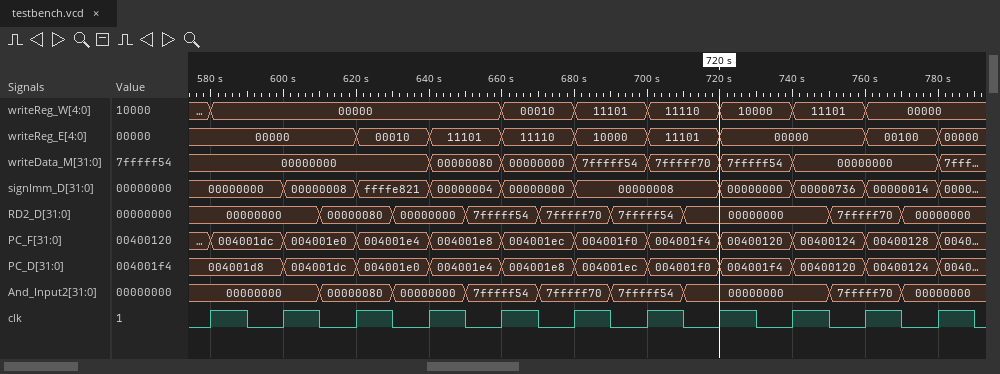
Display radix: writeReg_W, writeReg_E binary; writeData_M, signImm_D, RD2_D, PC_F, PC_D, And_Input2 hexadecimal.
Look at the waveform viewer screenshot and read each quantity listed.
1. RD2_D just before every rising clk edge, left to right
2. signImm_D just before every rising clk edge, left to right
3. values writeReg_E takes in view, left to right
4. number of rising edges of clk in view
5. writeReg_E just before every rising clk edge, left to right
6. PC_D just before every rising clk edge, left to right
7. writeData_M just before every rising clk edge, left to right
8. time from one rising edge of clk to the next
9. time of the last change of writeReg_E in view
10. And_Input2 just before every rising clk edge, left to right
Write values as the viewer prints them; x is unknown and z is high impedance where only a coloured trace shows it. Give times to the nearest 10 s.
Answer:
00000000, 00000000, 00000080, 00000000, 7fffff54, 7fffff70, 7fffff54, 00000000, 00000000, 7fffff70, 00000000
00000000, 00000000, 00000008, ffffe821, 00000004, 00000000, 00000008, 00000008, 00000000, 00000736, 00000014
00000, 00010, 11101, 11110, 10000, 11101, 00000, 00100, 00000
11
00000, 00000, 00000, 00010, 11101, 11110, 10000, 11101, 00000, 00000, 00100
004001d8, 004001d8, 004001dc, 004001e0, 004001e4, 004001e8, 004001ec, 004001f0, 004001f4, 00400120, 00400124
00000000, 00000000, 00000000, 00000000, 00000080, 00000000, 7fffff54, 7fffff70, 7fffff54, 00000000, 00000000
20 s
780 s
00000000, 00000000, 00000080, 00000000, 7fffff54, 7fffff70, 7fffff54, 00000000, 00000000, 7fffff70, 00000000
